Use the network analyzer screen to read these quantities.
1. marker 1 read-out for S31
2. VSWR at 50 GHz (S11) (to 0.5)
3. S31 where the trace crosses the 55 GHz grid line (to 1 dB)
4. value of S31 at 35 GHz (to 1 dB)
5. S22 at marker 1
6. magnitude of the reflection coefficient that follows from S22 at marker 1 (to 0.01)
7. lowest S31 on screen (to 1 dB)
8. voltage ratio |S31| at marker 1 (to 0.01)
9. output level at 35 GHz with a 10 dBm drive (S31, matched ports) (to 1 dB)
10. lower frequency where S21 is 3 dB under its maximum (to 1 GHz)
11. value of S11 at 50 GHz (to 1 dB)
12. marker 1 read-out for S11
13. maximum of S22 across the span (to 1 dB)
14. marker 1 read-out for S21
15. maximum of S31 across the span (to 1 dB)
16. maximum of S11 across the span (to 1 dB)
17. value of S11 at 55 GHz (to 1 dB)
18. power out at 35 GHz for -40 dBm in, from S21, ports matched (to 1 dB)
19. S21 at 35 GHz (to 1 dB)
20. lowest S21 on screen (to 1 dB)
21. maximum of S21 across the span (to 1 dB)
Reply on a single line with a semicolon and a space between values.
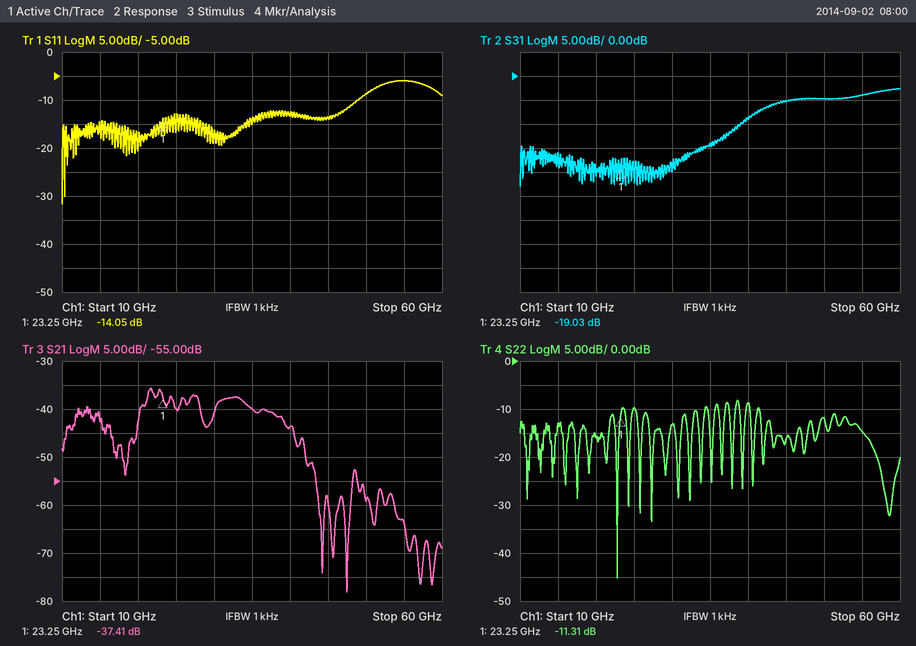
-19.03 dB; 2.0; -4 dB; -14 dB; -11.31 dB; 0.27; -23 dB; 0.11; -4 dBm; 21 GHz; -9 dB; -14.05 dB; -8 dB; -37.41 dB; -3 dB; -6 dB; -6 dB; -80 dBm; -40 dB; -78 dB; -36 dB
